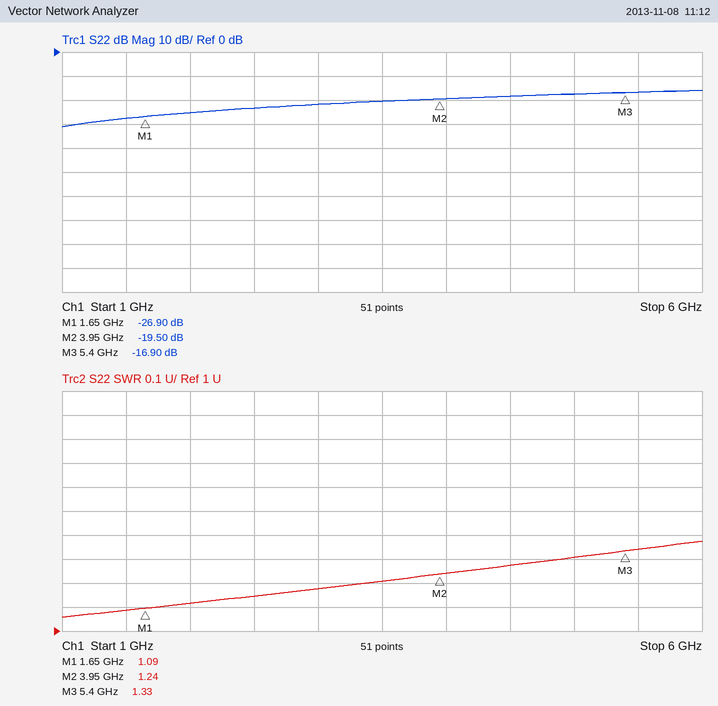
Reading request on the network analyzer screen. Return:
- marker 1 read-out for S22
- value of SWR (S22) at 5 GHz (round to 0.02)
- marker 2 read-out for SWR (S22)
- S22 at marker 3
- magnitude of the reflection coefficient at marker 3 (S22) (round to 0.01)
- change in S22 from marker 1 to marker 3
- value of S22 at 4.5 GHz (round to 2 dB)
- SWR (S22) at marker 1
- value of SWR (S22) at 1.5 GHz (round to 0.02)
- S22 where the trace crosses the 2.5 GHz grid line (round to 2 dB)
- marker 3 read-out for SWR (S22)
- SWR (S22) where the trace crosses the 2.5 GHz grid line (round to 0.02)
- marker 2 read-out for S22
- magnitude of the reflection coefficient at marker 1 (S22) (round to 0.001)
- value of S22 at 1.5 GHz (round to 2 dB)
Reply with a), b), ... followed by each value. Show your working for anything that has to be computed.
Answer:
a) -26.90 dB
b) 1.30
c) 1.24
d) -16.90 dB
e) 10^(-16.9/20) ≈ 0.14
f) -16.9 − (-26.9) = 10.00 dB
g) -18 dB
h) 1.09
i) 1.08
j) -24 dB
k) 1.33
l) 1.14
m) -19.50 dB
n) 10^(-26.9/20) ≈ 0.045
o) -28 dB
